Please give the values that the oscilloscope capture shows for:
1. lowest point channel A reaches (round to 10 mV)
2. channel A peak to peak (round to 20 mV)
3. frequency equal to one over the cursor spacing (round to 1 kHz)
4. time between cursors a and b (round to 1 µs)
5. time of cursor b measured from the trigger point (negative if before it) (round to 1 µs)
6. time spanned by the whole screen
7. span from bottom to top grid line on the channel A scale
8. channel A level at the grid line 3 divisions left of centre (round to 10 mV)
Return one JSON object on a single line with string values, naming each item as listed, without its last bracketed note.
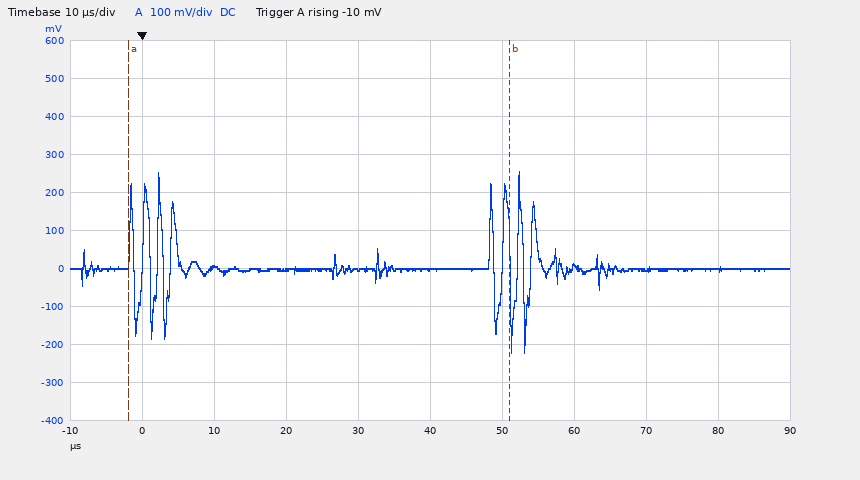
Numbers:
{"lowest point channel A reaches": "-220 mV", "channel A peak to peak": "480 mV", "frequency equal to one over the cursor spacing": "19 kHz", "time between cursors a and b": "53 µs", "time of cursor b measured from the trigger point (negative if before it)": "+51 µs", "time spanned by the whole screen": "100 µs", "span from bottom to top grid line on the channel A scale": "1 V", "channel A level at the grid line 3 divisions left of centre": "0 mV"}
